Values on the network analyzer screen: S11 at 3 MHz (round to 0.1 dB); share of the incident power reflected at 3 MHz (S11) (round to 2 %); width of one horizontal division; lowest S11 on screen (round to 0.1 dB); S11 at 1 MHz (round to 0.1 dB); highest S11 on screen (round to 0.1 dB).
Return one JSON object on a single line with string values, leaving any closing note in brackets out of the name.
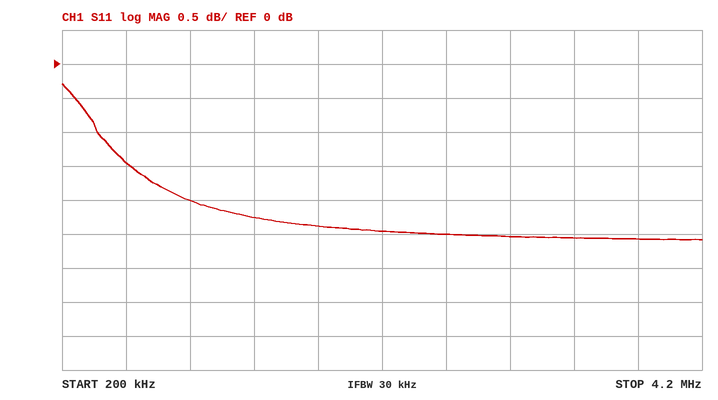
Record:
{"S11 at 3 MHz": "-2.5 dB", "share of the incident power reflected at 3 MHz (S11)": "56 %", "width of one horizontal division": "400 kHz", "lowest S11 on screen": "-2.6 dB", "S11 at 1 MHz": "-2.0 dB", "highest S11 on screen": "-0.3 dB"}
